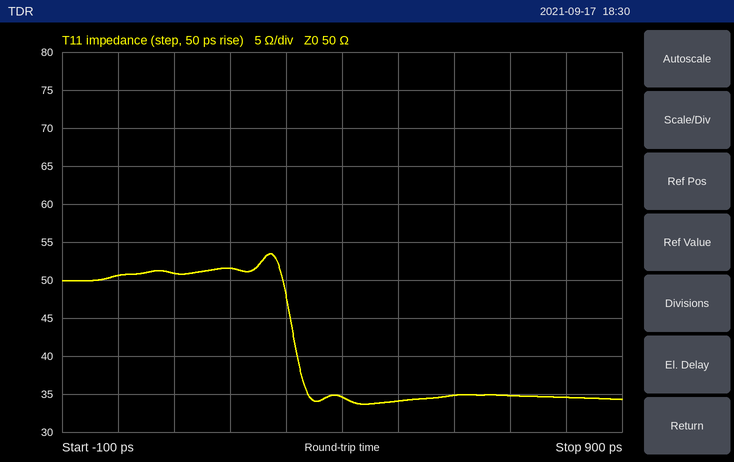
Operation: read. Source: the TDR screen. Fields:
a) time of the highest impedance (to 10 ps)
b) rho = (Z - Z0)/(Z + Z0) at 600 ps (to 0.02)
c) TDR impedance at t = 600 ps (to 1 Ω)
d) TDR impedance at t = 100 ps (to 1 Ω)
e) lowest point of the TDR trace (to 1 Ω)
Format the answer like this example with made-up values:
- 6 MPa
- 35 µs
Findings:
- 270 ps
- -0.18
- 35 Ω
- 51 Ω
- 34 Ω
